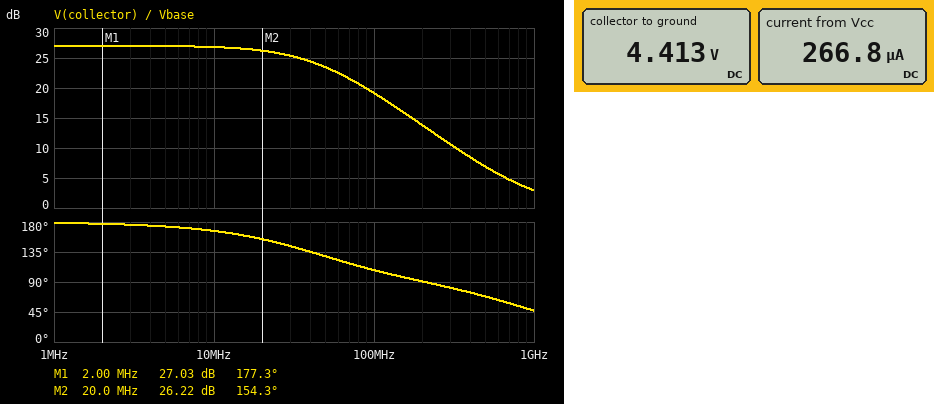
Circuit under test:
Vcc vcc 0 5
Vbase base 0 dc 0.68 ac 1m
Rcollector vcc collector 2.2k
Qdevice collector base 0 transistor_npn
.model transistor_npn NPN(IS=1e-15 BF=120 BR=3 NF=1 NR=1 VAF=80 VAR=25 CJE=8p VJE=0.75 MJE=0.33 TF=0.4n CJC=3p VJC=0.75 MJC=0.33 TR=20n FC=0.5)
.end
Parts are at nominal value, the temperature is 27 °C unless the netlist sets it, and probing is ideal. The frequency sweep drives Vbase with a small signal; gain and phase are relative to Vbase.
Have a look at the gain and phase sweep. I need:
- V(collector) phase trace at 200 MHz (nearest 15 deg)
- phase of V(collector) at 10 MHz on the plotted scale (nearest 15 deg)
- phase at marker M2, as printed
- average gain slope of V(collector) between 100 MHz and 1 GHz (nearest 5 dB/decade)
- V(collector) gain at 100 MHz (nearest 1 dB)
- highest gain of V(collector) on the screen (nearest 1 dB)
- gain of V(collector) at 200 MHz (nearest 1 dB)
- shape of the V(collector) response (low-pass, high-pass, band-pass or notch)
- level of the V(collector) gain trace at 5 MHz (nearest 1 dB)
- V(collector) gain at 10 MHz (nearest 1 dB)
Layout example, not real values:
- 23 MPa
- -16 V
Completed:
- 90 deg
- 165 deg
- 154.3 deg
- -15 dB/decade
- 19 dB
- 27 dB
- 14 dB
- low-pass
- 27 dB
- 27 dB
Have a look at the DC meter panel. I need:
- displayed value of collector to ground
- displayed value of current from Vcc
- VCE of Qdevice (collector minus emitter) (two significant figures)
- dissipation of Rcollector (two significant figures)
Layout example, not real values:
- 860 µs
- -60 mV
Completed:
- 4.413 V
- 266.8 µA
- 4.4 V
- 160 µW
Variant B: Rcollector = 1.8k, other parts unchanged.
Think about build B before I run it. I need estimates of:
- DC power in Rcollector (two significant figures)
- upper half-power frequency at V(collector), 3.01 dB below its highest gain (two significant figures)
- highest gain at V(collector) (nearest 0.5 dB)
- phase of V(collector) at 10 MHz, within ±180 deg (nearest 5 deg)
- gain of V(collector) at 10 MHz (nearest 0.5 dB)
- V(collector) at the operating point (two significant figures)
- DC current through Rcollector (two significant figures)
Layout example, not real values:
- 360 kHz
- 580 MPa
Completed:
- 130 µW
- 54 MHz
- 25.5 dB
- 170 deg
- 25.0 dB
- 4.5 V
- 270 µA
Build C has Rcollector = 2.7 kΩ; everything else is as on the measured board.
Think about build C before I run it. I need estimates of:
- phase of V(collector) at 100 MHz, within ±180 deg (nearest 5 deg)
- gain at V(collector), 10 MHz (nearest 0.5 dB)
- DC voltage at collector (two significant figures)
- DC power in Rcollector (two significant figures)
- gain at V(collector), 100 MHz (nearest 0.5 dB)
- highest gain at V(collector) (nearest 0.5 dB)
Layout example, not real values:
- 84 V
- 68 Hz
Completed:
- 105 deg
- 28.5 dB
- 4.3 V
- 190 µW
- 19.5 dB
- 29.0 dB
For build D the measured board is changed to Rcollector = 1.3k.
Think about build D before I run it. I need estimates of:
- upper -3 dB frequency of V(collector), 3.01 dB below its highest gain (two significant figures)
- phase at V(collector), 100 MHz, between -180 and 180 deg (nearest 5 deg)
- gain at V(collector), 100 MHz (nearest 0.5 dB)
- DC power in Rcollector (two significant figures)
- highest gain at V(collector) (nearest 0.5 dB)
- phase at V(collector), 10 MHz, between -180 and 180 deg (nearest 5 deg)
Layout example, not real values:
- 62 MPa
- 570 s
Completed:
- 76 MHz
- 120 deg
- 18.0 dB
- 93 µW
- 22.5 dB
- 170 deg
